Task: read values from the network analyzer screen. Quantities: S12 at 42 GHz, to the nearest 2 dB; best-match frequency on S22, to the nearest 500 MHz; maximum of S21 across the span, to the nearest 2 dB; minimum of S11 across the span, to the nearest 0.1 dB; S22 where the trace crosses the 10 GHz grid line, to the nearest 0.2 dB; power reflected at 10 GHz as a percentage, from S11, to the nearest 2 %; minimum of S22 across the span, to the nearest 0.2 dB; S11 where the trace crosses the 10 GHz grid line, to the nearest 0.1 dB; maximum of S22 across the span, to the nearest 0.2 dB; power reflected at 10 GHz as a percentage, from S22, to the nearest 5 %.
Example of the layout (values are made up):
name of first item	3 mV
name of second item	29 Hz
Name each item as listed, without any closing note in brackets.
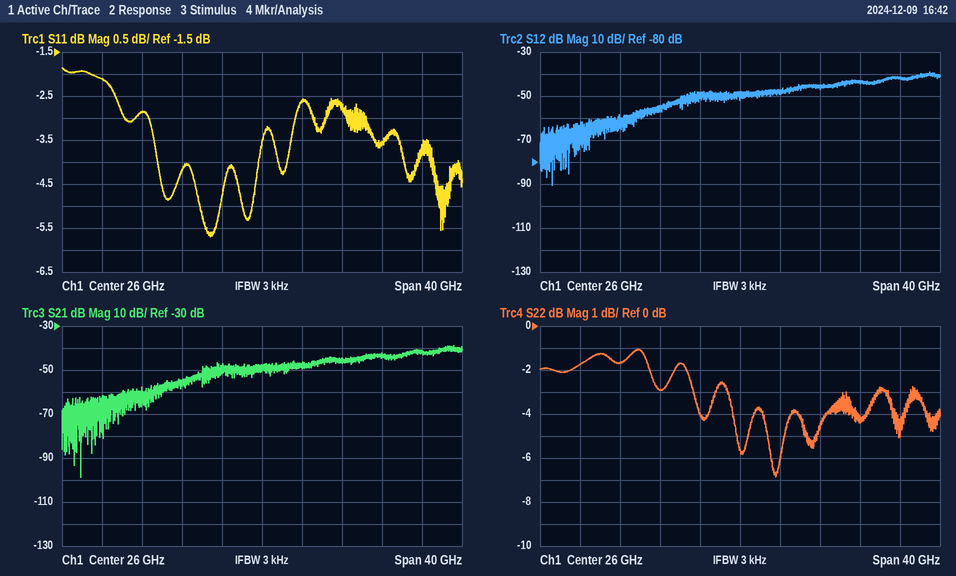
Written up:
S12 at 42 GHz, to the nearest 2 dB	-42 dB
best-match frequency on S22, to the nearest 500 MHz	29.5 GHz
maximum of S21 across the span, to the nearest 2 dB	-38 dB
minimum of S11 across the span, to the nearest 0.1 dB	-5.7 dB
S22 where the trace crosses the 10 GHz grid line, to the nearest 0.2 dB	-1.8 dB
power reflected at 10 GHz as a percentage, from S11, to the nearest 2 %	62 %
minimum of S22 across the span, to the nearest 0.2 dB	-6.8 dB
S11 where the trace crosses the 10 GHz grid line, to the nearest 0.1 dB	-2.1 dB
maximum of S22 across the span, to the nearest 0.2 dB	-1.0 dB
power reflected at 10 GHz as a percentage, from S22, to the nearest 5 %	65 %
